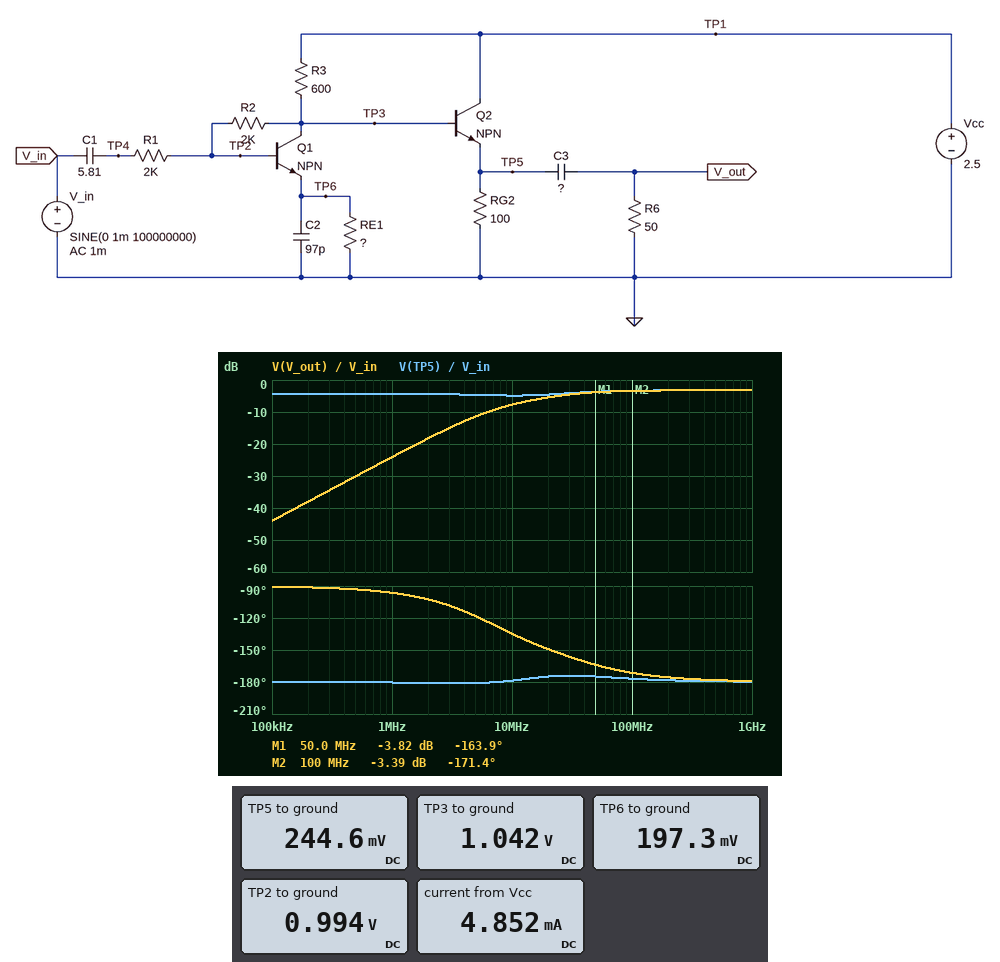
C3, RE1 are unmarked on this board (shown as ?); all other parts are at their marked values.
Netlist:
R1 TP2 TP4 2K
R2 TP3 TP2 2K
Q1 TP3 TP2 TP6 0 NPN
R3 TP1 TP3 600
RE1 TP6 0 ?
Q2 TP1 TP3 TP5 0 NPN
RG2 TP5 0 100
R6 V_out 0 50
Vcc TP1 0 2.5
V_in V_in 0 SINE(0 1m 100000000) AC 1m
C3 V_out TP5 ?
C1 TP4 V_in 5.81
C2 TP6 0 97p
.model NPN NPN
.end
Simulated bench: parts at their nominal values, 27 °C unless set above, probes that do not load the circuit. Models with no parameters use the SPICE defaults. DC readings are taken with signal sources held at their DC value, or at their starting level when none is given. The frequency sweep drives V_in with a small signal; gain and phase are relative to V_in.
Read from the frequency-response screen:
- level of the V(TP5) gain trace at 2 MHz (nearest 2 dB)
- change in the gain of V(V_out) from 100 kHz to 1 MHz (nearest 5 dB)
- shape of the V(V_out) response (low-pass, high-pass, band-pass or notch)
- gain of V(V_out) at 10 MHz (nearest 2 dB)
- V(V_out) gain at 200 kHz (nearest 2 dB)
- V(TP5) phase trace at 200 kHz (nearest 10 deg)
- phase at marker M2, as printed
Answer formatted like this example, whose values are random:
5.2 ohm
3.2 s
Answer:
-4 dB
20 dB
high-pass
-8 dB
-38 dB
-180 deg
-171.4 deg
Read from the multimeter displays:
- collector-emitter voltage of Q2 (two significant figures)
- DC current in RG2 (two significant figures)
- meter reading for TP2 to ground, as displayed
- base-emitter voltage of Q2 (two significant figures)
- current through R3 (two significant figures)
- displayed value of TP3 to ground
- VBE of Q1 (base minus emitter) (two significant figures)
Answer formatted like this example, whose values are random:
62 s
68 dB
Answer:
2.3 V
2.4 mA
0.994 V
800 mV
2.4 mA
1.042 V
800 mV
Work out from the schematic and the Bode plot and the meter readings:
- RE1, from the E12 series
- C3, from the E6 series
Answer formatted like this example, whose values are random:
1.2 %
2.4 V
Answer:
82 Ω
330 pF
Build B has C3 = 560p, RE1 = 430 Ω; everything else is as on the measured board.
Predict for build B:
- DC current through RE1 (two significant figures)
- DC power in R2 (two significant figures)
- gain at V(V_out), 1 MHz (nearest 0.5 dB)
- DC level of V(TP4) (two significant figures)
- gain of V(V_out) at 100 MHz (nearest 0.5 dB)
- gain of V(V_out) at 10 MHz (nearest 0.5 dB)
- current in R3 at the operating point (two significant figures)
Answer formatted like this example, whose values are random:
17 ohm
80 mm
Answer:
1.6 mA
500 nW
-26.5 dB
1.5 V
-2.0 dB
-6.0 dB
1.7 mA
